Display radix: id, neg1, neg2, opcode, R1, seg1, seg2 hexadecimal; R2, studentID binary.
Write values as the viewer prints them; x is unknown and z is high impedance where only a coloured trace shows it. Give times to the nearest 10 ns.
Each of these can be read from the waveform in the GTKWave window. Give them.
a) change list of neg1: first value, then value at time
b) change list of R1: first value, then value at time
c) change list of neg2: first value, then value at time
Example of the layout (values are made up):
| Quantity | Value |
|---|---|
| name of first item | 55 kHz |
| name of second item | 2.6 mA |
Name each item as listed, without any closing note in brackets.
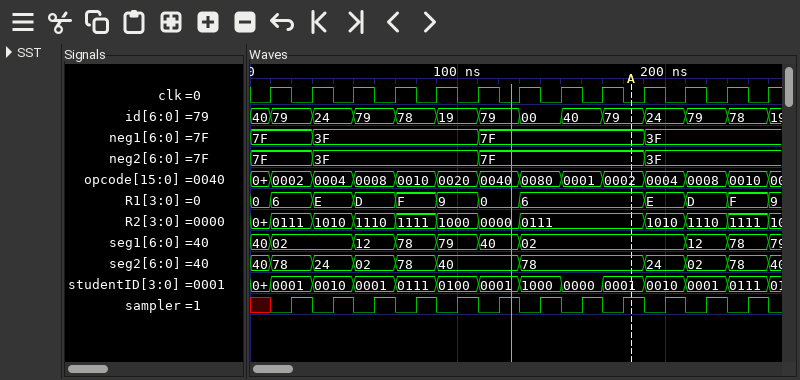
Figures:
| Quantity | Value |
|---|---|
| change list of neg1: first value, then value at time | 7F, 3F at 30 ns, 7F at 110 ns, 3F at 190 ns |
| change list of R1: first value, then value at time | 0, 6 at 10 ns, E at 30 ns, D at 50 ns, F at 70 ns, 9 at 90 ns, 0 at 110 ns, 6 at 130 ns, E at 190 ns, D at 210 ns, F at 230 ns, 9 at 250 ns |
| change list of neg2: first value, then value at time | 7F, 3F at 30 ns, 7F at 110 ns, 3F at 190 ns |
